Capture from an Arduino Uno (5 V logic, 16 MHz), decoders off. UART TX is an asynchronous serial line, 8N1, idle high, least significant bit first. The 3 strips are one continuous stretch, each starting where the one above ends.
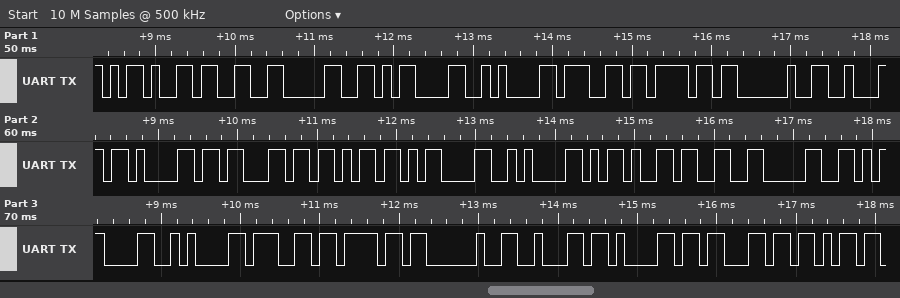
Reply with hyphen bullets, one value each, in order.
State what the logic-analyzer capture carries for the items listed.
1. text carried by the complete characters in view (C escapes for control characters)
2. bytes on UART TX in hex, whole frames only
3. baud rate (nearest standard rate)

- "-30\r\ngo back\r\n-30\r\ngo back"
- 2D 33 30 0D 0A 67 6F 20 62 61 63 6B 0D 0A 2D 33 30 0D 0A 67 6F 20 62 61 63 6B
- 9600 baud
